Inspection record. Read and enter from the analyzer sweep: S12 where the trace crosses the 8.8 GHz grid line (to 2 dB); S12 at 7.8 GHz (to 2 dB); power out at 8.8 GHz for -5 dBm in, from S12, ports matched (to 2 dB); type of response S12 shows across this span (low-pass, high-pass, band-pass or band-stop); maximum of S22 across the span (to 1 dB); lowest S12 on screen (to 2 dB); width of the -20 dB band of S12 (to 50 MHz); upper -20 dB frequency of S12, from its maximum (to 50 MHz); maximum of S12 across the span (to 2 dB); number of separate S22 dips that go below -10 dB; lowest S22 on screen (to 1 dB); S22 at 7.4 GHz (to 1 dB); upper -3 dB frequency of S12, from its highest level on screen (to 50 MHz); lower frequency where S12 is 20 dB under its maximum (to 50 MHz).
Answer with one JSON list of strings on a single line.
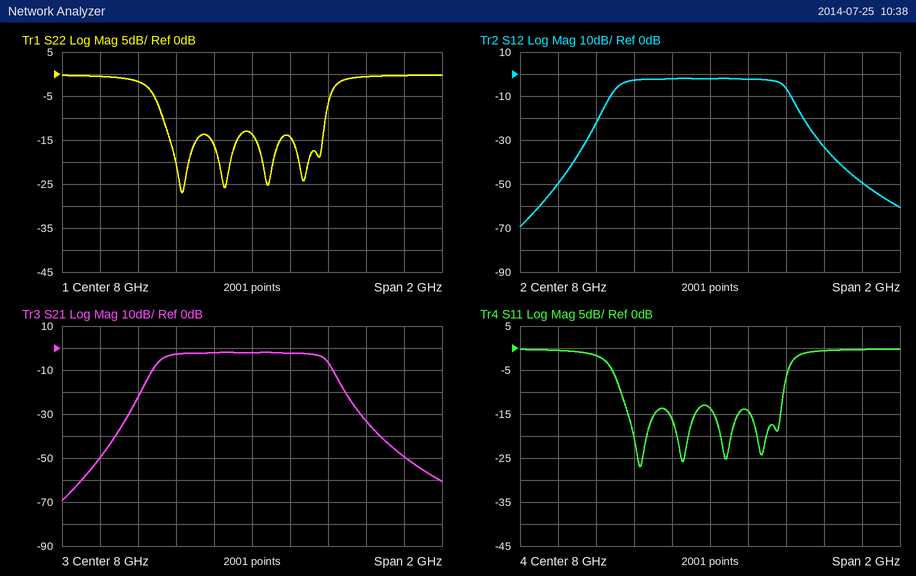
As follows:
["-50 dB", "-2 dB", "-54 dBm", "band-pass", "0 dB", "-70 dB", "1.10 GHz", "8.50 GHz", "-2 dB", "4", "-27 dB", "-2 dB", "8.40 GHz", "7.40 GHz"]
